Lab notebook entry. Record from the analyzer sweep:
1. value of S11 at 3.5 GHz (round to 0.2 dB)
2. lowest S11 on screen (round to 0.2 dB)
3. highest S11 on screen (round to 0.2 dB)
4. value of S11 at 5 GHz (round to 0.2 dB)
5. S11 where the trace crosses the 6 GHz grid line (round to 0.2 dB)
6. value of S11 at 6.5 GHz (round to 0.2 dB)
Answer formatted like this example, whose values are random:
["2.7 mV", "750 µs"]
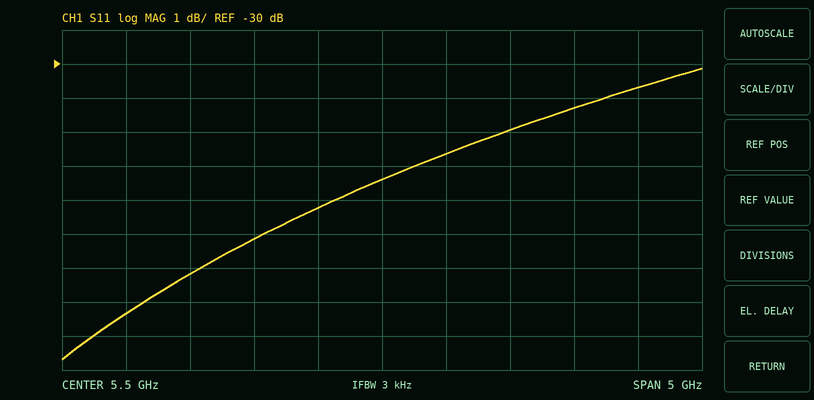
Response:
["-37.4 dB", "-38.6 dB", "-30.2 dB", "-34.2 dB", "-32.6 dB", "-32.0 dB"]
